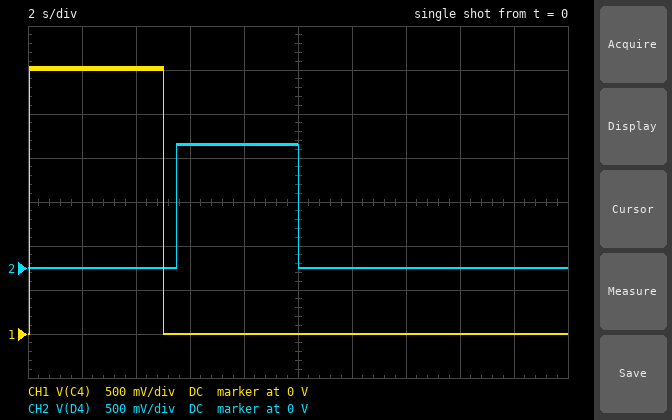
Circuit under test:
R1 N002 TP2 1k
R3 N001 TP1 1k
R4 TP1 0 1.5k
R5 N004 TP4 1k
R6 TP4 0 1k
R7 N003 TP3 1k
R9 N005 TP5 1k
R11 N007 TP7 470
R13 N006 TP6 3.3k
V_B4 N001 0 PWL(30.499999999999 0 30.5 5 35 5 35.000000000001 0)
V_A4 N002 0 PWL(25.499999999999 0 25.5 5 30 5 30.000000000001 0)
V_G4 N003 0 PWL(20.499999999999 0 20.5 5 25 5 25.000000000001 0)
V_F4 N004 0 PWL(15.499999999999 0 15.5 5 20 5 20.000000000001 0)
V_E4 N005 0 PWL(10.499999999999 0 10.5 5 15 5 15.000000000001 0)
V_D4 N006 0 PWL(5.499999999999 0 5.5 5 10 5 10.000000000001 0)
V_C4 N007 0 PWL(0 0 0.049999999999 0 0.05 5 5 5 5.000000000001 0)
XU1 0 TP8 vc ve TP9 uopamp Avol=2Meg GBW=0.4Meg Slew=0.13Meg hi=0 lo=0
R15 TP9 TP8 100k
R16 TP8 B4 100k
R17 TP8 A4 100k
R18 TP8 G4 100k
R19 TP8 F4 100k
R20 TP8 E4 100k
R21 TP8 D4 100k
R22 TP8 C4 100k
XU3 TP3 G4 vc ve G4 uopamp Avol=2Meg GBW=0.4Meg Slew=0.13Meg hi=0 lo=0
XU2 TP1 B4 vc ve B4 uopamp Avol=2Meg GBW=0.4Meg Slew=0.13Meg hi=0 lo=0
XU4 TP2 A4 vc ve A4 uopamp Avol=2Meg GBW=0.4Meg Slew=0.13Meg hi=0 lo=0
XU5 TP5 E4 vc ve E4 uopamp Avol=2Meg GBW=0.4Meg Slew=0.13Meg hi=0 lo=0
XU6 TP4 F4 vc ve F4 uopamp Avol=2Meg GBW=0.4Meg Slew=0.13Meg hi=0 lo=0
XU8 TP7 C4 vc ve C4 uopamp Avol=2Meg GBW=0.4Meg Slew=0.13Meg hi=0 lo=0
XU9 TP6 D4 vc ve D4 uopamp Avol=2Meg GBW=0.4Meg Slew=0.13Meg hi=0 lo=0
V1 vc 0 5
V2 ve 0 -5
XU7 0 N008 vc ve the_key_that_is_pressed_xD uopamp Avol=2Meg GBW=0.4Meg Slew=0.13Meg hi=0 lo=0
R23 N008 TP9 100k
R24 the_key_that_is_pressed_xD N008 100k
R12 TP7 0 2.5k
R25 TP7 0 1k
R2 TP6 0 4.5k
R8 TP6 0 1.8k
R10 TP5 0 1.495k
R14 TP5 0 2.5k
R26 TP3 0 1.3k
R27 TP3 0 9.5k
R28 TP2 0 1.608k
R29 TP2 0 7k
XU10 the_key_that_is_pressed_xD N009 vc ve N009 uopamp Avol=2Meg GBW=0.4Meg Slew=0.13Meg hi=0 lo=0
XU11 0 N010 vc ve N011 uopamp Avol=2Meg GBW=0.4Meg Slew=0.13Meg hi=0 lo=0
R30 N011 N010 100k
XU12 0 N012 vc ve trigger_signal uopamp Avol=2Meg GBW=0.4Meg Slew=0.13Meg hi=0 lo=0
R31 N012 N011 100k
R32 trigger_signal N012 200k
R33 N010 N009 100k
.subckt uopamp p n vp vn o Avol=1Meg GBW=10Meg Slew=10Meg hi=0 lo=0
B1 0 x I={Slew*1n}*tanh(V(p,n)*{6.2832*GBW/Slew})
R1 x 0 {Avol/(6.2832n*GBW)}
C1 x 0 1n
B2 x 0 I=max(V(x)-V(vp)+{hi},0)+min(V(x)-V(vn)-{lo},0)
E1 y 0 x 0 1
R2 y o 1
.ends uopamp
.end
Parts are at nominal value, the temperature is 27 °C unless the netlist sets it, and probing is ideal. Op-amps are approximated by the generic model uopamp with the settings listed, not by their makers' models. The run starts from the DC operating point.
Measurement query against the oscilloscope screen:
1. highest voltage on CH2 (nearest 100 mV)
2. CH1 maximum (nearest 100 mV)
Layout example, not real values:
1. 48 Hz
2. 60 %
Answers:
1. 1.4 V
2. 3.0 V
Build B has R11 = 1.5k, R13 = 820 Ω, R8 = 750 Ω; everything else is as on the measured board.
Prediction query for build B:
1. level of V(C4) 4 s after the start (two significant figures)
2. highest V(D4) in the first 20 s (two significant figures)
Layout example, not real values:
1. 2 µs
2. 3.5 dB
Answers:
1. 1.6 V
2. 2.2 V
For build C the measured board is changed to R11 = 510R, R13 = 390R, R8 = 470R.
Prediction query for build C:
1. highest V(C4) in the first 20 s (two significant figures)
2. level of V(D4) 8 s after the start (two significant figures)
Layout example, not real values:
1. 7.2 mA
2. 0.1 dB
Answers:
1. 2.9 V
2. 2.6 V
